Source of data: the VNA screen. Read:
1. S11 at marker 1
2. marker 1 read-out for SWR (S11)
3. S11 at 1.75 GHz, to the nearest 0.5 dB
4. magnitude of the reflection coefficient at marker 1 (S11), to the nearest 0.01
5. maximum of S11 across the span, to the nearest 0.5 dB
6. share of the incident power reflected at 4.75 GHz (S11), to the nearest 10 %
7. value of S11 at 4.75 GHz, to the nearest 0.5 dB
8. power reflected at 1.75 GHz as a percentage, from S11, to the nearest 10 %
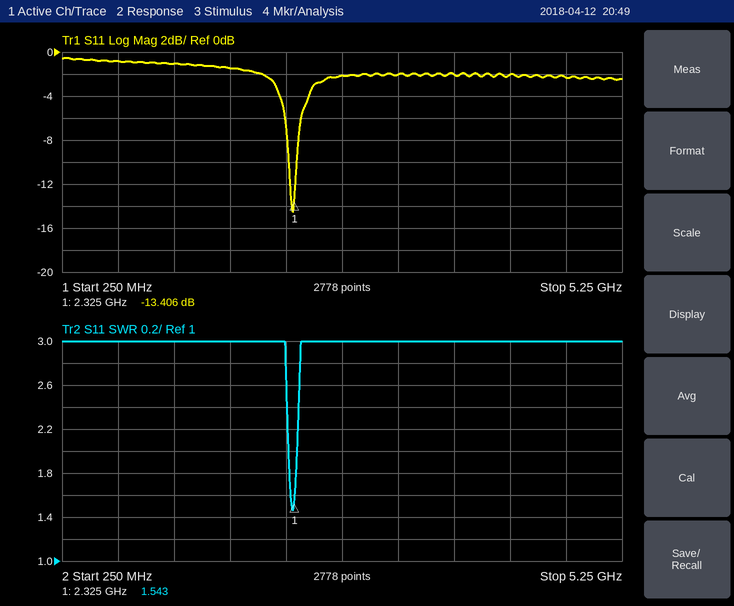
-13.406 dB
1.543
-1.5 dB
0.21
-0.5 dB
60 %
-2.5 dB
70 %
